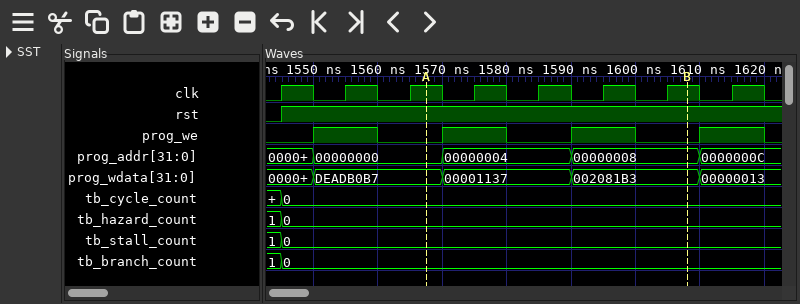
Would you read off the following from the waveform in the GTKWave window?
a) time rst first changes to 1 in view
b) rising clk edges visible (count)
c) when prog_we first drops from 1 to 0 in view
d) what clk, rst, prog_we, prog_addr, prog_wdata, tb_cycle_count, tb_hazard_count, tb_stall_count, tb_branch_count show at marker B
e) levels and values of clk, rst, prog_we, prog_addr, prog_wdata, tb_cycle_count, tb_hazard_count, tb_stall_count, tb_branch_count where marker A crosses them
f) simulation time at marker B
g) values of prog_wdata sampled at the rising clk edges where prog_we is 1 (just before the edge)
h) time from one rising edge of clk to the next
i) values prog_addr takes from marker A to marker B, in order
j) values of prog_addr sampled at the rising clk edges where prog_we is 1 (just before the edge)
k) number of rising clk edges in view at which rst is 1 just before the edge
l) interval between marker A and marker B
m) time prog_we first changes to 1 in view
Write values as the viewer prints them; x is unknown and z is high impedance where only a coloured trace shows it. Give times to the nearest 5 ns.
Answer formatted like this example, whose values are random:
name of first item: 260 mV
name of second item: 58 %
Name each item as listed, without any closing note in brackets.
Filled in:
time rst first changes to 1 in view: 1545 ns
rising clk edges visible: 8
when prog_we first drops from 1 to 0 in view: 1560 ns
what clk, rst, prog_we, prog_addr, prog_wdata, tb_cycle_count, tb_hazard_count, tb_stall_count, tb_branch_count show at marker B: clk=1, rst=1, prog_we=0, prog_addr=00000008, prog_wdata=002081B3, tb_cycle_count=0, tb_hazard_count=0, tb_stall_count=0, tb_branch_count=0
levels and values of clk, rst, prog_we, prog_addr, prog_wdata, tb_cycle_count, tb_hazard_count, tb_stall_count, tb_branch_count where marker A crosses them: clk=1, rst=1, prog_we=0, prog_addr=00000000, prog_wdata=DEADB0B7, tb_cycle_count=0, tb_hazard_count=0, tb_stall_count=0, tb_branch_count=0
simulation time at marker B: 1610 ns
values of prog_wdata sampled at the rising clk edges where prog_we is 1: DEADB0B7, 00001137, 002081B3, 00000013
time from one rising edge of clk to the next: 10 ns
values prog_addr takes from marker A to marker B, in order: 00000000, 00000004, 00000008
values of prog_addr sampled at the rising clk edges where prog_we is 1: 00000000, 00000004, 00000008, 0000000C
number of rising clk edges in view at which rst is 1 just before the edge: 7
interval between marker A and marker B: 40 ns
time prog_we first changes to 1 in view: 1550 ns
